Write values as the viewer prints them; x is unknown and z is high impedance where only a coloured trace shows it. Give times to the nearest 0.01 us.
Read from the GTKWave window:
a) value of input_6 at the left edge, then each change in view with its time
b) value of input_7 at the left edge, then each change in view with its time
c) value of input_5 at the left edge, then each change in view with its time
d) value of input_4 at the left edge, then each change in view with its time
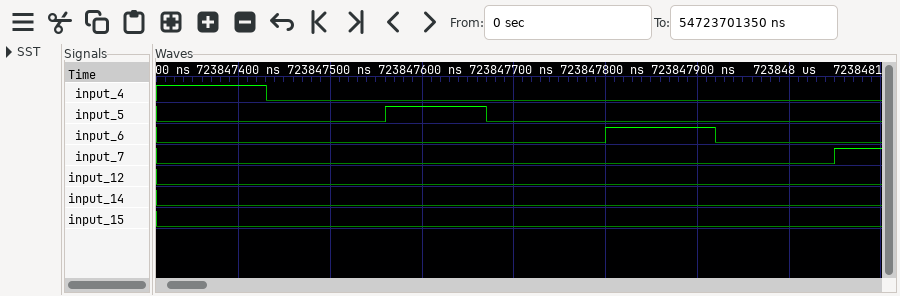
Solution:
0, 1 at 723847.8 us, 0 at 723847.92 us
0, 1 at 723848.05 us
0, 1 at 723847.56 us, 0 at 723847.67 us
1, 0 at 723847.43 us
